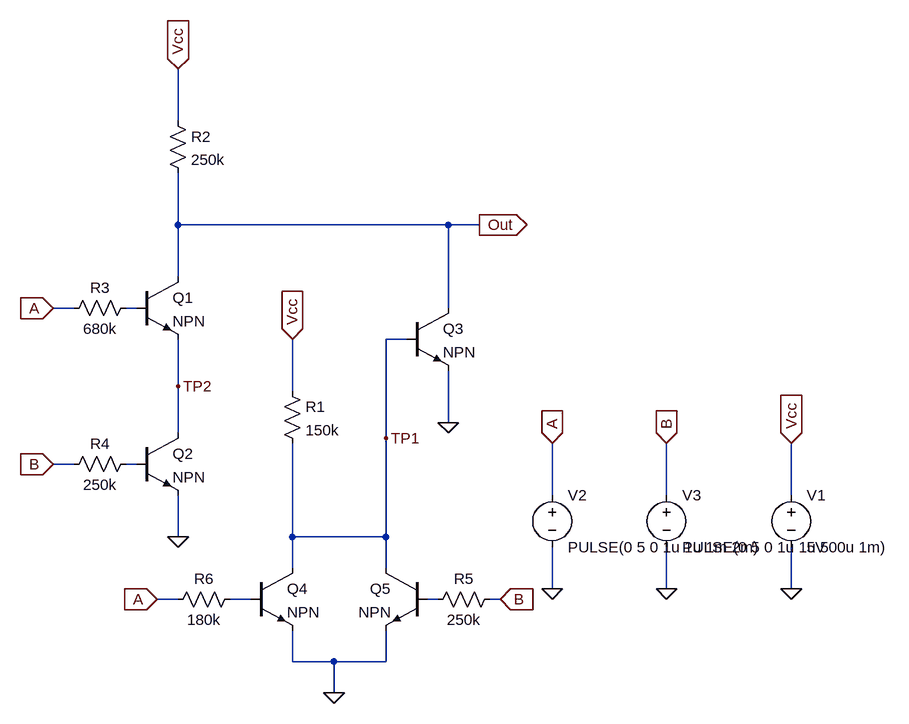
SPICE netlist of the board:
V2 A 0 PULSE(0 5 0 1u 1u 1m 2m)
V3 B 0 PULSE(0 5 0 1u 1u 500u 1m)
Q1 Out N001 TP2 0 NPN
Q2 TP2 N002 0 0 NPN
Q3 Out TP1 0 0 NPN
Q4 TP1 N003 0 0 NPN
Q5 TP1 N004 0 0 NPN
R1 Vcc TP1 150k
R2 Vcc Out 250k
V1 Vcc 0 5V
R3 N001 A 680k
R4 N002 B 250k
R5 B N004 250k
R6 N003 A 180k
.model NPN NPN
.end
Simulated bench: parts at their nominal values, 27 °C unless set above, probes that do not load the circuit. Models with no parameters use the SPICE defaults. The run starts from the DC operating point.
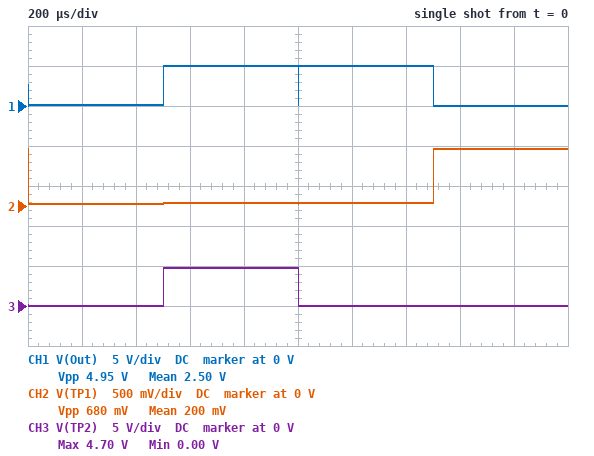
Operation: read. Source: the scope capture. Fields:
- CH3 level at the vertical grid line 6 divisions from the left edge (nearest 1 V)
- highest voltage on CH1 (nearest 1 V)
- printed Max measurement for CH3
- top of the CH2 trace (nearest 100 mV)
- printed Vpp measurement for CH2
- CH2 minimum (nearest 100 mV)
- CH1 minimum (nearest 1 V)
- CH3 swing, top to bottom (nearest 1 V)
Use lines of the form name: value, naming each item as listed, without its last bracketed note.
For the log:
CH3 level at the vertical grid line 6 divisions from the left edge: 0 V
highest voltage on CH1: 5 V
printed Max measurement for CH3: 4.70 V
top of the CH2 trace: 700 mV
printed Vpp measurement for CH2: 680 mV
CH2 minimum: 0 V
CH1 minimum: 0 V
CH3 swing, top to bottom: 5 V
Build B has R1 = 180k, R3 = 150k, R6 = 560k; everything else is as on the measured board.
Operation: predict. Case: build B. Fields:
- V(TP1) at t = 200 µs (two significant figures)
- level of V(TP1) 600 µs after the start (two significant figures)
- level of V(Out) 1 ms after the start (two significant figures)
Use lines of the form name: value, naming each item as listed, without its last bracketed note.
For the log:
V(TP1) at t = 200 µs: 30 mV
level of V(TP1) 600 µs after the start: 45 mV
level of V(Out) 1 ms after the start: 5.0 V
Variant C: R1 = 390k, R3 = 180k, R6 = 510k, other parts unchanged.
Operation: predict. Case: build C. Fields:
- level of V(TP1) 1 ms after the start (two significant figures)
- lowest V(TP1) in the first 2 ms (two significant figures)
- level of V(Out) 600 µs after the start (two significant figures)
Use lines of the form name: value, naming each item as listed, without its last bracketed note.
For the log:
level of V(TP1) 1 ms after the start: 33 mV
lowest V(TP1) in the first 2 ms: 24 mV
level of V(Out) 600 µs after the start: 5.0 V
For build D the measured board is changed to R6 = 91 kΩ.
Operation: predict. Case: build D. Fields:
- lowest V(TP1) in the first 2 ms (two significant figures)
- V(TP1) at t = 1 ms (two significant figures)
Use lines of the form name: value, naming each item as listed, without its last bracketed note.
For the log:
lowest V(TP1) in the first 2 ms: 24 mV
V(TP1) at t = 1 ms: 26 mV
